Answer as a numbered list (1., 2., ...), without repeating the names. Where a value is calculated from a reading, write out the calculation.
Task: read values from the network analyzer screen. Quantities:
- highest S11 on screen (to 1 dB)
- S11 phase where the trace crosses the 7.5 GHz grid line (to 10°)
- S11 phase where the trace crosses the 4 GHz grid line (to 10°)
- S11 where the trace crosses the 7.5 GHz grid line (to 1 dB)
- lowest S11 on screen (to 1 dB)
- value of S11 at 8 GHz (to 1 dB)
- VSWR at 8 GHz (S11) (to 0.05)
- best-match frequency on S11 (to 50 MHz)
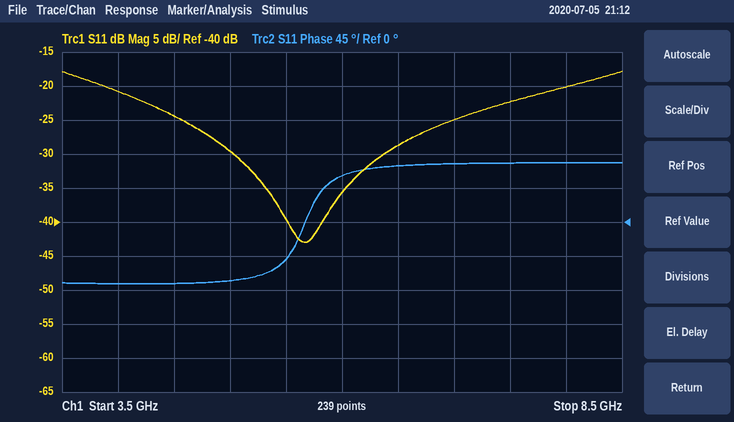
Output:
1. -18 dB
2. 80°
3. -80°
4. -22 dB
5. -43 dB
6. -20 dB
7. |Γ| = 10^(-20/20) = 0.1000; VSWR = (1 + 0.1000)/(1 − 0.1000) ≈ 1.22, so 1.20 to the nearest 0.05
8. 5.65 GHz
